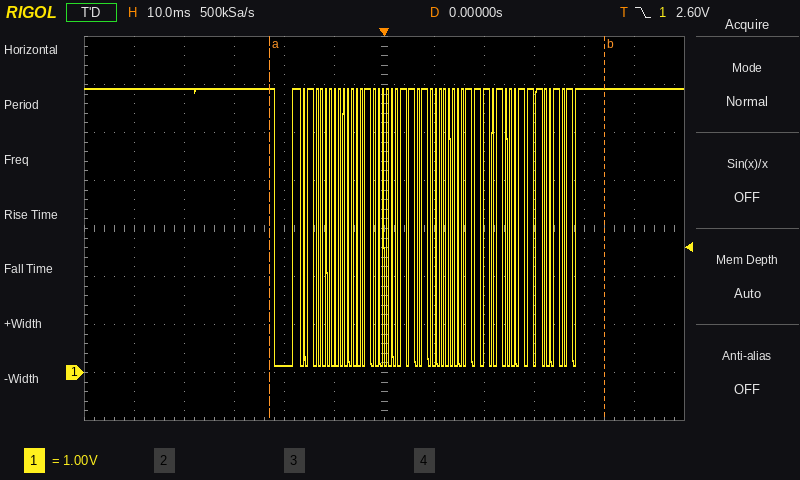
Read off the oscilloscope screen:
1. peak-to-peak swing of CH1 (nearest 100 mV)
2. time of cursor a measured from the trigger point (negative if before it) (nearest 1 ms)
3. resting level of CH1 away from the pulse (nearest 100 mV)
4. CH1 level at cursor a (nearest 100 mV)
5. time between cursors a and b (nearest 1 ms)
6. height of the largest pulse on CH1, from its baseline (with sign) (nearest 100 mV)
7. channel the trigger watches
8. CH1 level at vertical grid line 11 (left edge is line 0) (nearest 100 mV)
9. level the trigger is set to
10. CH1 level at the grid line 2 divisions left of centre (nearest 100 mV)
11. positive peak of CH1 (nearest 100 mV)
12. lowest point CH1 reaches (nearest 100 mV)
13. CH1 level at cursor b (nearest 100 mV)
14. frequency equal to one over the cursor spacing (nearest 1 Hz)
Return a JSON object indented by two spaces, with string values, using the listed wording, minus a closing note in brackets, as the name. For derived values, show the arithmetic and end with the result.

{
  "peak-to-peak swing of CH1": "5.9 V − (100 mV) = 5.8 V",
  "time of cursor a measured from the trigger point (negative if before it)": "-23 ms",
  "resting level of CH1 away from the pulse": "5.9 V",
  "CH1 level at cursor a": "5.9 V",
  "time between cursors a and b": "67 ms",
  "height of the largest pulse on CH1, from its baseline (with sign)": "100 mV − (5.9 V) = -5.8 V",
  "channel the trigger watches": "CH1",
  "CH1 level at vertical grid line 11 (left edge is line 0)": "5.9 V",
  "level the trigger is set to": "2.60 V",
  "CH1 level at the grid line 2 divisions left of centre": "100 mV",
  "positive peak of CH1": "5.9 V",
  "lowest point CH1 reaches": "100 mV",
  "CH1 level at cursor b": "5.9 V",
  "frequency equal to one over the cursor spacing": "1 / 67 ms ≈ 15 Hz"
}
